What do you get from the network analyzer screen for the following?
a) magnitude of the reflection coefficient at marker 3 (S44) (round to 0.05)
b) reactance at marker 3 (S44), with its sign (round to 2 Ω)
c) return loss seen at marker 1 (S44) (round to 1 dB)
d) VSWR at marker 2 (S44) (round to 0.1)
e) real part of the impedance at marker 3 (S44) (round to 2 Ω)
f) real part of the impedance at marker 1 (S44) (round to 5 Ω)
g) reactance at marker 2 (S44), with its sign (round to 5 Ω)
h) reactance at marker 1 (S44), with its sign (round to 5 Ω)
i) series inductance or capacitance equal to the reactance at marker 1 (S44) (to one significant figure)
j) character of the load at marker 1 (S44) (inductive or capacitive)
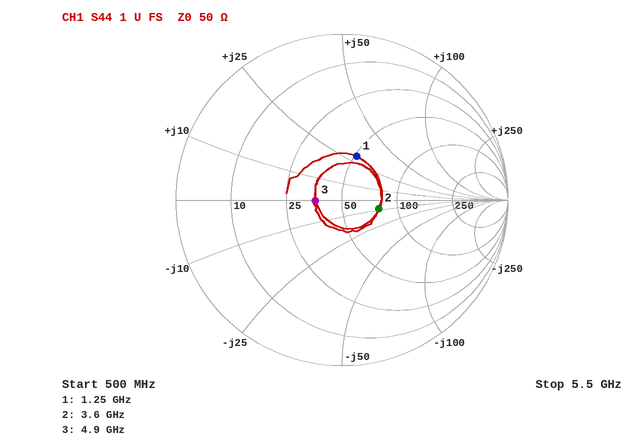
0.15
0 Ω
11 dB
1.6
36 Ω
50 Ω
-10 Ω
+30 Ω
4 nH
inductive
